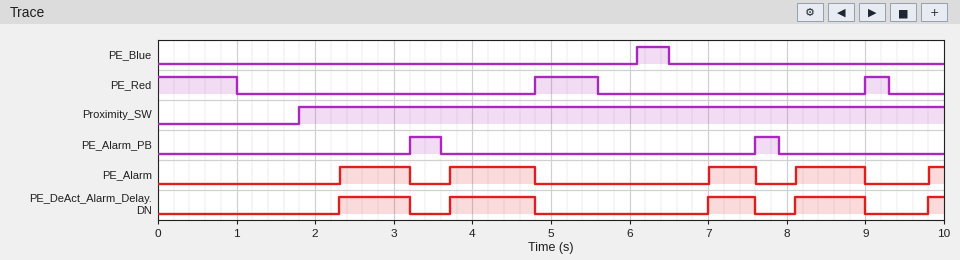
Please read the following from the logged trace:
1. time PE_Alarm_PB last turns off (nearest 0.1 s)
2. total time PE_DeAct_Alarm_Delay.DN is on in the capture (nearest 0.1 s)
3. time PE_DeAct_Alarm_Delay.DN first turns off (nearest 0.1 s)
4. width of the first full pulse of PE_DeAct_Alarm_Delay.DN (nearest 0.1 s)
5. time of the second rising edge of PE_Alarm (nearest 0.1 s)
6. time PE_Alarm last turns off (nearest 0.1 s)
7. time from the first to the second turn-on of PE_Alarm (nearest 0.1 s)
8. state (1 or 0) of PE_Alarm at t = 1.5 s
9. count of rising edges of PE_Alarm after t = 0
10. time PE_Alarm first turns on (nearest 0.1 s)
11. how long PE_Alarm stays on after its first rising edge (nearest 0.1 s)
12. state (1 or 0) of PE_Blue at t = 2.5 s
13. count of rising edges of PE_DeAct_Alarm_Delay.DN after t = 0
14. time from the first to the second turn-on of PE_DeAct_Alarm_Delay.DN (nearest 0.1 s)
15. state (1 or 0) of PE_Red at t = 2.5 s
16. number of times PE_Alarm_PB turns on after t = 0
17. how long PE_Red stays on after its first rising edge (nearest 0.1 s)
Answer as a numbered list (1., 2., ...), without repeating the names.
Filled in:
1. 7.9 s
2. 3.7 s
3. 3.2 s
4. 0.9 s
5. 3.7 s
6. 9.0 s
7. 1.4 s
8. 0
9. 5
10. 2.3 s
11. 0.9 s
12. 0
13. 5
14. 1.4 s
15. 0
16. 2
17. 0.8 s
